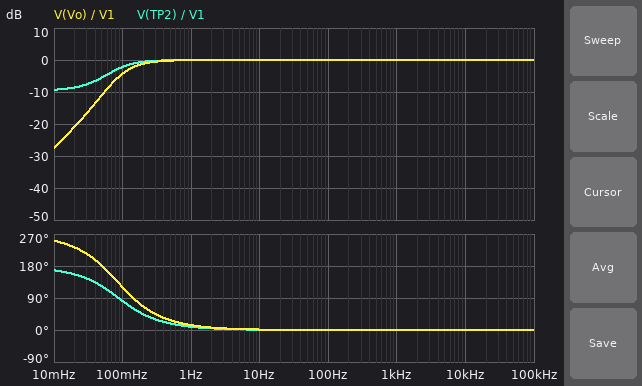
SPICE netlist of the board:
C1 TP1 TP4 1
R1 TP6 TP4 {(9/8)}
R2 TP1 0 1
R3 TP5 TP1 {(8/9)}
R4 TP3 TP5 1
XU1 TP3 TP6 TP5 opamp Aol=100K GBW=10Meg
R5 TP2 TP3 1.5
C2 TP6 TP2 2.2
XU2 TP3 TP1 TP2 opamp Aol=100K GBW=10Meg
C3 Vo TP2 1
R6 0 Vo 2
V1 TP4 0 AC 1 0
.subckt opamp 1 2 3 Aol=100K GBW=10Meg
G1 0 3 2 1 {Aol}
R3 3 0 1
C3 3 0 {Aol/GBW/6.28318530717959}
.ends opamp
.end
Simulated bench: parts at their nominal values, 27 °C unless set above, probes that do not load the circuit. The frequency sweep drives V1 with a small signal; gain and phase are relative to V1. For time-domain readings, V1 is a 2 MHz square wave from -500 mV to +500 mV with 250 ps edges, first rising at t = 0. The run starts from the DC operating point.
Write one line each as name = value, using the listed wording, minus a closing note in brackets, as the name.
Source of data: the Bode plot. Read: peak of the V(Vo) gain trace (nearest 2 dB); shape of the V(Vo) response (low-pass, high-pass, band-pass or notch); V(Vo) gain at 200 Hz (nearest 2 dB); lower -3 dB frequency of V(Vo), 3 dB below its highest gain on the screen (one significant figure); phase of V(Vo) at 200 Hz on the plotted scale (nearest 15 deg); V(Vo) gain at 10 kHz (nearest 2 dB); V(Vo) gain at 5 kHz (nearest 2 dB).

peak of the V(Vo) gain trace = 0 dB
shape of the V(Vo) response = high-pass
V(Vo) gain at 200 Hz = 0 dB
lower -3 dB frequency of V(Vo), 3 dB below its highest gain on the screen = 100 mHz
phase of V(Vo) at 200 Hz on the plotted scale = 0 deg
V(Vo) gain at 10 kHz = 0 dB
V(Vo) gain at 5 kHz = 0 dB
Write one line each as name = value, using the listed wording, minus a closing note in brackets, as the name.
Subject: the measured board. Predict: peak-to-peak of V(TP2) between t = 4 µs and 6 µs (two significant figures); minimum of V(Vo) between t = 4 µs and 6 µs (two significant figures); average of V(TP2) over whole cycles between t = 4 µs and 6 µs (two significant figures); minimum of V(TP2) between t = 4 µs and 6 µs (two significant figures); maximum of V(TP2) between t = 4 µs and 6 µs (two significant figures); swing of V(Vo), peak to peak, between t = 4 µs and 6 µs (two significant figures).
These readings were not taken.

peak-to-peak of V(TP2) between t = 4 µs and 6 µs = 1.5 V
minimum of V(Vo) between t = 4 µs and 6 µs = -230 mV
average of V(TP2) over whole cycles between t = 4 µs and 6 µs = 670 mV
minimum of V(TP2) between t = 4 µs and 6 µs = -64 mV
maximum of V(TP2) between t = 4 µs and 6 µs = 1.4 V
swing of V(Vo), peak to peak, between t = 4 µs and 6 µs = 1.5 V
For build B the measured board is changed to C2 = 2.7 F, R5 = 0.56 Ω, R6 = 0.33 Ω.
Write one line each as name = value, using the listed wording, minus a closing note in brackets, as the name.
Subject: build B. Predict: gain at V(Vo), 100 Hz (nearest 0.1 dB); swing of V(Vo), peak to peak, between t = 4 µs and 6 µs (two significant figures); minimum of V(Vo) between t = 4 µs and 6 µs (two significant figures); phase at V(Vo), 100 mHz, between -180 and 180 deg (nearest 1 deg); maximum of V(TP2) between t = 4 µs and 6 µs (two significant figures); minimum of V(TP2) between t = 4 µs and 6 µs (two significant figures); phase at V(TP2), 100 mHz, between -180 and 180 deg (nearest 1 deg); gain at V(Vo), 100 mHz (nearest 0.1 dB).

gain at V(Vo), 100 Hz = 0 dB
swing of V(Vo), peak to peak, between t = 4 µs and 6 µs = 1.3 V
minimum of V(Vo) between t = 4 µs and 6 µs = -170 mV
phase at V(Vo), 100 mHz, between -180 and 180 deg = -169 deg
maximum of V(TP2) between t = 4 µs and 6 µs = 920 mV
minimum of V(TP2) between t = 4 µs and 6 µs = -420 mV
phase at V(TP2), 100 mHz, between -180 and 180 deg = 113 deg
gain at V(Vo), 100 mHz = -34.6 dB
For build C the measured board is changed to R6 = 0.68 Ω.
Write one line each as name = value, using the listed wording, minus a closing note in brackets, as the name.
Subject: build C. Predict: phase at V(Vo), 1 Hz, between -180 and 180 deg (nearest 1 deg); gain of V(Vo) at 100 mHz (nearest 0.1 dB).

phase at V(Vo), 1 Hz, between -180 and 180 deg = 22 deg
gain of V(Vo) at 100 mHz = -10.3 dB
